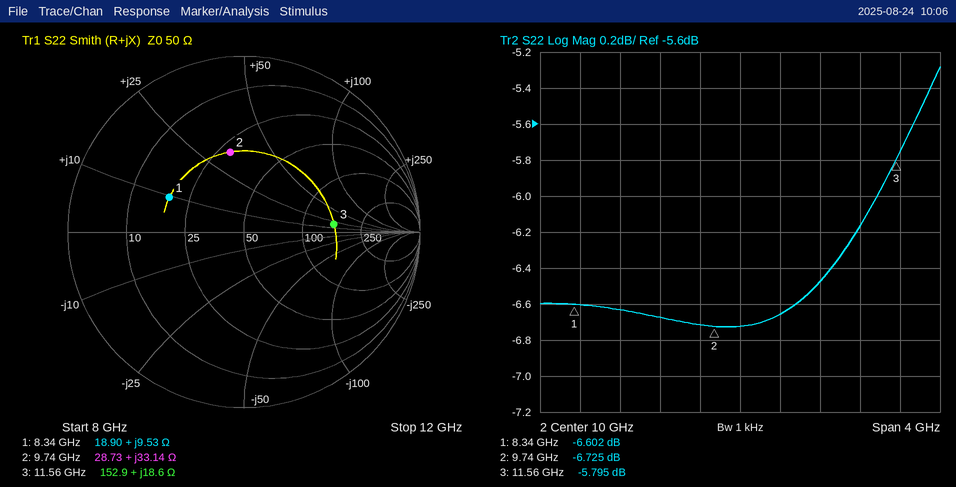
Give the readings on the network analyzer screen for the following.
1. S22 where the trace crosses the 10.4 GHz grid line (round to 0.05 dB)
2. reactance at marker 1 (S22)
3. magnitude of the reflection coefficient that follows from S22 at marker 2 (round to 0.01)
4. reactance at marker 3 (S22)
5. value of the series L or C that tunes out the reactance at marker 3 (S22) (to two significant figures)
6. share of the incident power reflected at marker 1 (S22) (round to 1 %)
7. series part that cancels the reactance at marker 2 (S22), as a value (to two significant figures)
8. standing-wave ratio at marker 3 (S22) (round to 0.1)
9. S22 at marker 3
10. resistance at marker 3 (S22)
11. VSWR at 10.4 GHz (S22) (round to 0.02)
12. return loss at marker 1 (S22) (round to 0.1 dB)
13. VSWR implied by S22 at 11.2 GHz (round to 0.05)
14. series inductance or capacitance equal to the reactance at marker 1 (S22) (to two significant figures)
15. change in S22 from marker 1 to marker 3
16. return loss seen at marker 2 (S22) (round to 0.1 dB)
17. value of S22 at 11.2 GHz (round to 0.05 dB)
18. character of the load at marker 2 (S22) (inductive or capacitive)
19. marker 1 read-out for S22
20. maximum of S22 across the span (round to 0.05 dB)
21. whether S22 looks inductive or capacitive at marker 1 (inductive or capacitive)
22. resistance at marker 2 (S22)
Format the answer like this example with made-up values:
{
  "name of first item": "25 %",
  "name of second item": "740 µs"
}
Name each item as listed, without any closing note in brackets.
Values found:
{
  "S22 where the trace crosses the 10.4 GHz grid line": "-6.65 dB",
  "reactance at marker 1": "+9.53 Ω",
  "magnitude of the reflection coefficient that follows from S22 at marker 2": "0.46",
  "reactance at marker 3": "+18.6 Ω",
  "value of the series L or C that tunes out the reactance at marker 3 (S22)": "740 fF",
  "share of the incident power reflected at marker 1 (S22)": "22 %",
  "series part that cancels the reactance at marker 2 (S22), as a value": "490 fF",
  "standing-wave ratio at marker 3 (S22)": "3.1",
  "S22 at marker 3": "-5.795 dB",
  "resistance at marker 3": "152.9 Ω",
  "VSWR at 10.4 GHz (S22)": "2.74",
  "return loss at marker 1 (S22)": "6.6 dB",
  "VSWR implied by S22 at 11.2 GHz": "2.95",
  "series inductance or capacitance equal to the reactance at marker 1 (S22)": "180 pH",
  "change in S22 from marker 1 to marker 3": "0.807 dB",
  "return loss seen at marker 2 (S22)": "6.7 dB",
  "value of S22 at 11.2 GHz": "-6.15 dB",
  "character of the load at marker 2 (S22)": "inductive",
  "marker 1 read-out for S22": "-6.602 dB",
  "maximum of S22 across the span": "-5.30 dB",
  "whether S22 looks inductive or capacitive at marker 1": "inductive",
  "resistance at marker 2": "28.73 Ω"
}
